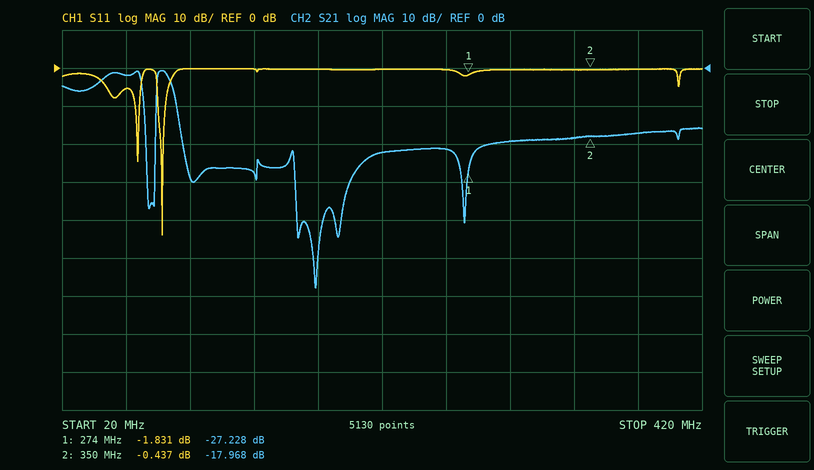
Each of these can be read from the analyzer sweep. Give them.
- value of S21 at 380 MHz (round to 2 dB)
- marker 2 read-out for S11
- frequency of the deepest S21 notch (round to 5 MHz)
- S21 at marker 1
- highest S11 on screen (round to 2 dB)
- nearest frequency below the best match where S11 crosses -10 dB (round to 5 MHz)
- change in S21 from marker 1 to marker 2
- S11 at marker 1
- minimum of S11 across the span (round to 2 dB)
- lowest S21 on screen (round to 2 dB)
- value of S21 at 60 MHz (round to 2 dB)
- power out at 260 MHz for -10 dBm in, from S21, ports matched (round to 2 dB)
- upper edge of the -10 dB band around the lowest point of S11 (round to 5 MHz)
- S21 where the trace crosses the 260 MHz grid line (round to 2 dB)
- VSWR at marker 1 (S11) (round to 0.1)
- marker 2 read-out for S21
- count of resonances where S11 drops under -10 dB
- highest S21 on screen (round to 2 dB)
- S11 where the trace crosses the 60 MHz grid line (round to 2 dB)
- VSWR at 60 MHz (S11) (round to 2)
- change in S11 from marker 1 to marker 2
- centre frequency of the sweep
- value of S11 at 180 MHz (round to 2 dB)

-18 dB
-0.437 dB
180 MHz
-27.228 dB
0 dB
80 MHz
9.260 dB
-1.831 dB
-44 dB
-58 dB
-2 dB
-32 dBm
85 MHz
-22 dB
9.5
-17.968 dB
2
0 dB
-6 dB
4
1.394 dB
220 MHz
0 dB
